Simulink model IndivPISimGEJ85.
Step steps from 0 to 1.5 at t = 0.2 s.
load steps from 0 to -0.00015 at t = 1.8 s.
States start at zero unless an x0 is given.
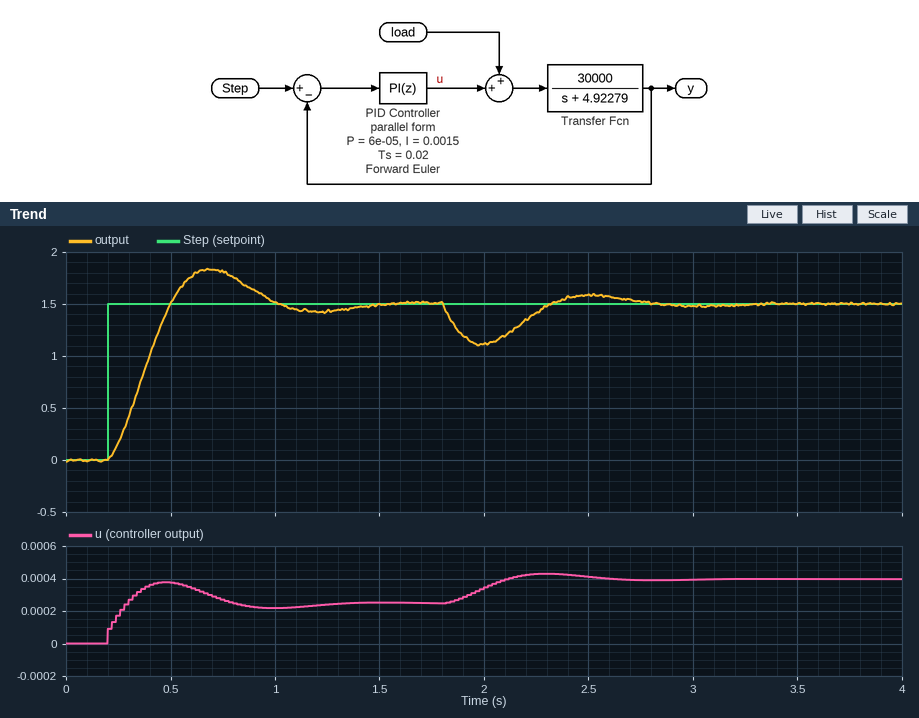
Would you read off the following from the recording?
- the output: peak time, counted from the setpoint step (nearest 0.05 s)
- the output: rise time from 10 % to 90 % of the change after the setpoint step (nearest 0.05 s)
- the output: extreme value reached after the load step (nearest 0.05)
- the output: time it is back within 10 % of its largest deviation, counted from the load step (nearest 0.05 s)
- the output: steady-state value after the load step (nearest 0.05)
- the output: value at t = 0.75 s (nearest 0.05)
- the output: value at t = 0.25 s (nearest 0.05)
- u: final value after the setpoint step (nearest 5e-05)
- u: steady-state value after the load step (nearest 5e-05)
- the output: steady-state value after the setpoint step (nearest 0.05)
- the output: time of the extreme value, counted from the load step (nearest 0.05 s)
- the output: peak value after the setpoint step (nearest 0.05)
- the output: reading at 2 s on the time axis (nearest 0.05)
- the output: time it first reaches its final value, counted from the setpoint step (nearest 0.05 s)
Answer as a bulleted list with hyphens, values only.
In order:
- 0.50 s
- 0.20 s
- 1.10
- 0.90 s
- 1.50
- 1.80
- 0.15
- 0.00025
- 0.00040
- 1.50
- 0.20 s
- 1.85
- 1.10
- 0.30 s
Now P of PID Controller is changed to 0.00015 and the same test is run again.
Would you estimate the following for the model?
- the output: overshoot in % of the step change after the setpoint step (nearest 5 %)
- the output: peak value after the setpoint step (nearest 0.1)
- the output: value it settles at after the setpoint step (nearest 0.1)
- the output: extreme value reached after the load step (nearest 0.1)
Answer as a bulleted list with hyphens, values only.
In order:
- 10 %
- 1.6
- 1.5
- 1.2
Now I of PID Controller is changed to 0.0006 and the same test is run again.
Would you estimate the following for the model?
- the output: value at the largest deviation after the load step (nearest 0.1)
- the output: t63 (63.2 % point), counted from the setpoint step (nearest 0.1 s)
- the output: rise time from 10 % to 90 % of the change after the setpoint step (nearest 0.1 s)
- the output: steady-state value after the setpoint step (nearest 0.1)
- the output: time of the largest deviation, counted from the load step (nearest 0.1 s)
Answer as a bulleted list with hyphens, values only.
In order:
- 1.0
- 0.3 s
- 0.5 s
- 1.5
- 0.3 s
